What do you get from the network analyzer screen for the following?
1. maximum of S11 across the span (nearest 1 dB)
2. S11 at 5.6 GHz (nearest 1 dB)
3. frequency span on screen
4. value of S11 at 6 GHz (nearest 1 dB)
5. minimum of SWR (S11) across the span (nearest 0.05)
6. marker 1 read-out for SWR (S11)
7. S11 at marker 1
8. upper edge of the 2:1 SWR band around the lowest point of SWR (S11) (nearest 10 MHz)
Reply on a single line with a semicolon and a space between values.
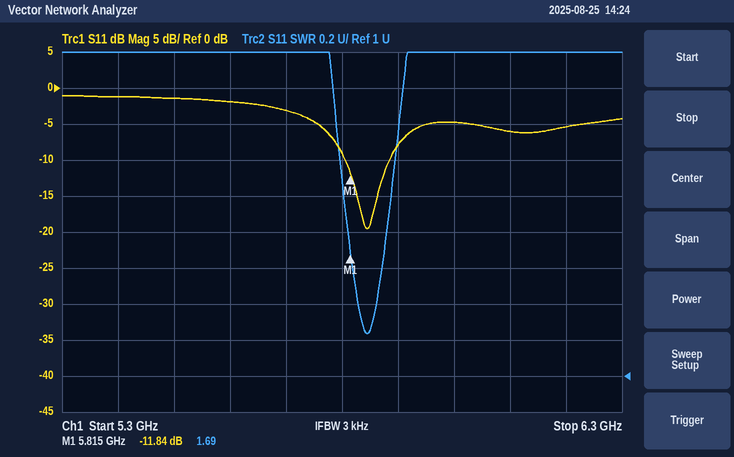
-1 dB; -2 dB; 1 GHz; -5 dB; 1.25; 1.69; -11.84 dB; 5.89 GHz
